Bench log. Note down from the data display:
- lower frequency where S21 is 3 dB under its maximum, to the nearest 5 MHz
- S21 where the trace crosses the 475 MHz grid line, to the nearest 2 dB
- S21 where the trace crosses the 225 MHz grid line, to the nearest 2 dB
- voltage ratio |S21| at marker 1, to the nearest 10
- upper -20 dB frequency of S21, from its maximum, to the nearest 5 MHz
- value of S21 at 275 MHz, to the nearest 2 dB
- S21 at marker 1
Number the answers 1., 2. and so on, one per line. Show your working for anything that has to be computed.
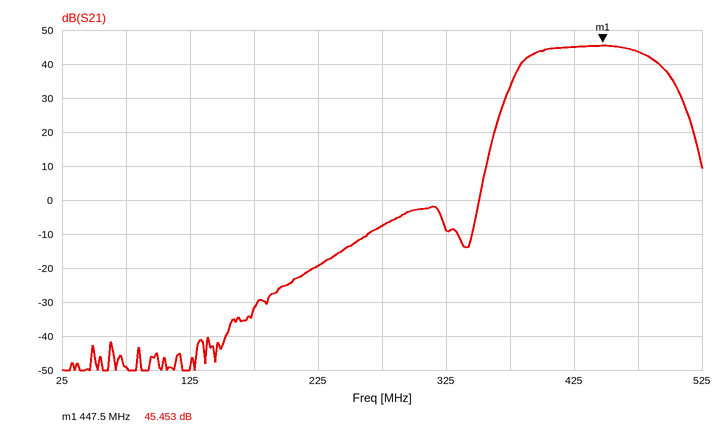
1. 390 MHz
2. 44 dB
3. -20 dB
4. 10^(45.453/20) ≈ 187, so 190 to the nearest 10
5. 515 MHz
6. -8 dB
7. 45.453 dB
